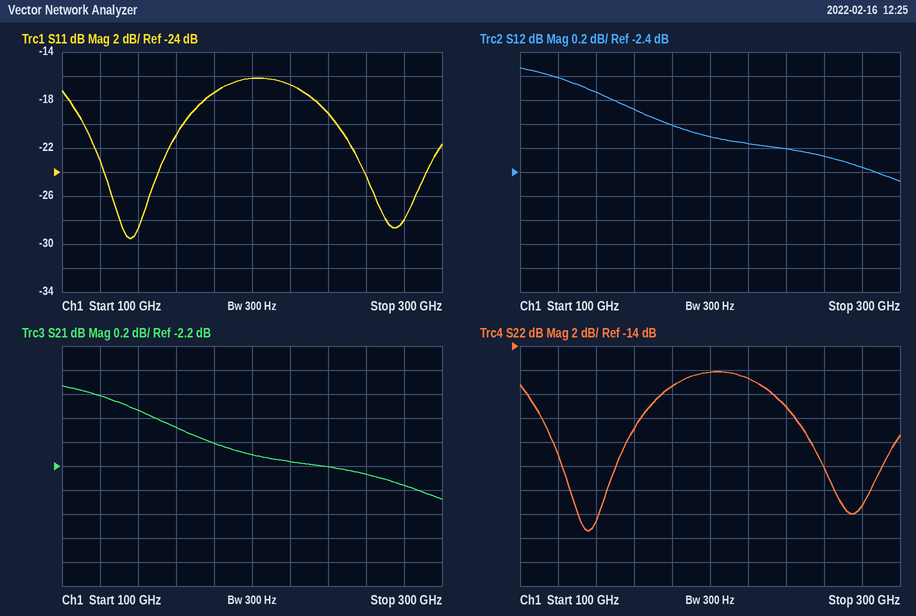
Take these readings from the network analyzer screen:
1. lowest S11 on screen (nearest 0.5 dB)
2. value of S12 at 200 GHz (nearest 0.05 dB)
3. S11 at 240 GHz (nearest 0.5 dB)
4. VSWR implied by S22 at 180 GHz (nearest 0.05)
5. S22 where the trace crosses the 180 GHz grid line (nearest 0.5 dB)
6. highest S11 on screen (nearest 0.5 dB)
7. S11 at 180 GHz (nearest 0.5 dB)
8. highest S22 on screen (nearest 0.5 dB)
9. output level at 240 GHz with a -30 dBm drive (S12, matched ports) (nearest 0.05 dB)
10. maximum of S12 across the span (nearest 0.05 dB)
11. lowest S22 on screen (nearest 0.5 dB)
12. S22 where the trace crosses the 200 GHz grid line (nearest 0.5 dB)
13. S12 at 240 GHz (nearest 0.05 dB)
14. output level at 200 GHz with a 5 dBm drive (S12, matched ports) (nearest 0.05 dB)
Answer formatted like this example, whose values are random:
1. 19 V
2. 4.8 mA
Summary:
1. -29.5 dB
2. -2.10 dB
3. -19.0 dB
4. 1.30
5. -17.5 dB
6. -16.0 dB
7. -17.5 dB
8. -16.0 dB
9. -32.20 dBm
10. -1.55 dB
11. -29.5 dB
12. -16.0 dB
13. -2.20 dB
14. 2.90 dBm
